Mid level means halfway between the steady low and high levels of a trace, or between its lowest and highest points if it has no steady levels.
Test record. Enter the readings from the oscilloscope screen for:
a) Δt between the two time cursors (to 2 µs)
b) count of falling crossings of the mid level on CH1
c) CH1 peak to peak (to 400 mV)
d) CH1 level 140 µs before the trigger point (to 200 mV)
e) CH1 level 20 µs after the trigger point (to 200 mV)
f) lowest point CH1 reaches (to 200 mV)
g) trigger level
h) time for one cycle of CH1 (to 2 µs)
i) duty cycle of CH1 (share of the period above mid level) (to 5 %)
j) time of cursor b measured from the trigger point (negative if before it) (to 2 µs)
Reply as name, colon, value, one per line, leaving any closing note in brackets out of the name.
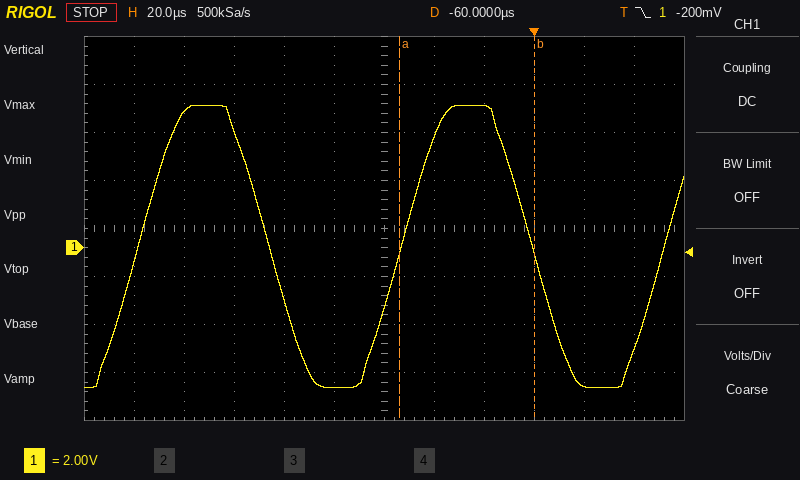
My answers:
Δt between the two time cursors: 54 µs
count of falling crossings of the mid level on CH1: 2
CH1 peak to peak: 11.6 V
CH1 level 140 µs before the trigger point: 5.6 V
CH1 level 20 µs after the trigger point: -5.8 V
lowest point CH1 reaches: -5.8 V
trigger level: -200 mV
time for one cycle of CH1: 106 µs
duty cycle of CH1 (share of the period above mid level): 50 %
time of cursor b measured from the trigger point (negative if before it): 0 µs
